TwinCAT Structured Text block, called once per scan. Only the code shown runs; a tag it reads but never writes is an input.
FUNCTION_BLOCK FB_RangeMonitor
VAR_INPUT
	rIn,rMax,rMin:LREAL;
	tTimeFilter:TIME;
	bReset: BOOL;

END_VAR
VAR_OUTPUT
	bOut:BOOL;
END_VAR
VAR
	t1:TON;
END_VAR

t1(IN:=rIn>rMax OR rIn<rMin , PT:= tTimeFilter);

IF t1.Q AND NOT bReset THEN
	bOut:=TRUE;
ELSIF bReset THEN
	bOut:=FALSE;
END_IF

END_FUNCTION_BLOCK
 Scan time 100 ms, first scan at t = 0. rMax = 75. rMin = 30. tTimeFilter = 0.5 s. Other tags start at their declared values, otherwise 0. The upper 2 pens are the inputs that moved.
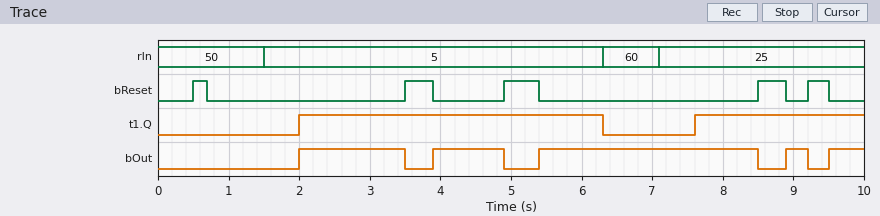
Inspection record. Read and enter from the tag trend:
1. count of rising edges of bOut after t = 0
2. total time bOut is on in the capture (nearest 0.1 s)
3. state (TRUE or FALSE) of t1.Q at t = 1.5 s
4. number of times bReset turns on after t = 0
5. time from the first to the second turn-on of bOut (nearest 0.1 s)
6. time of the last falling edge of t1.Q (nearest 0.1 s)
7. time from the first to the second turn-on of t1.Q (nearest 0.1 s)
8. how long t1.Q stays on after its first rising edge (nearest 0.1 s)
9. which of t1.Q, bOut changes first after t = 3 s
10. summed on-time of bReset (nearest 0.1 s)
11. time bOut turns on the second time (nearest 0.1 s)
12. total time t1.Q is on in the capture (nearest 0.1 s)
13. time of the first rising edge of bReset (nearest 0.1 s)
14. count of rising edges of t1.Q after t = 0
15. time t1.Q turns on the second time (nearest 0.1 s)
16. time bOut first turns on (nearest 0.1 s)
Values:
5
6.4 s
FALSE
5
1.9 s
6.3 s
5.6 s
4.3 s
bOut
1.8 s
3.9 s
6.7 s
0.5 s
2
7.6 s
2.0 s
